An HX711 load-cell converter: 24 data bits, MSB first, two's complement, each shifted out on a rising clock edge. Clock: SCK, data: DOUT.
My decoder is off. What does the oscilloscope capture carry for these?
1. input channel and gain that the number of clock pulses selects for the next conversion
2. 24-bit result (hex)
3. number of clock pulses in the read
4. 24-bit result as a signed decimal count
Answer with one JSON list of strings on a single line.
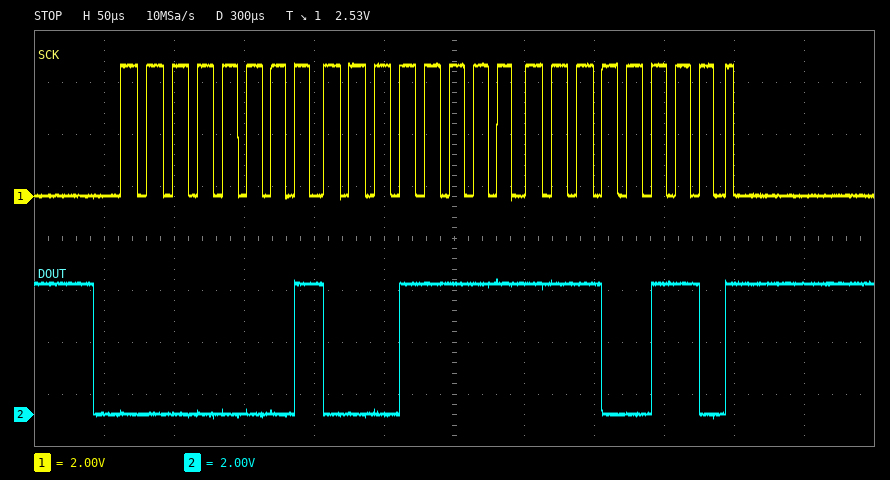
["channel A, gain 128", "0x011FE6", "25", "73702"]
